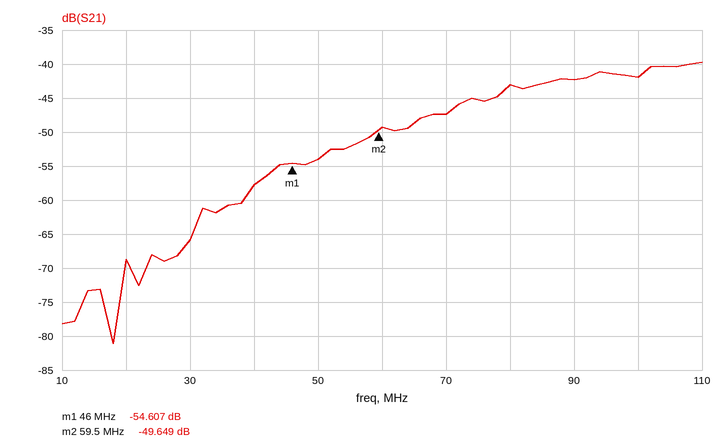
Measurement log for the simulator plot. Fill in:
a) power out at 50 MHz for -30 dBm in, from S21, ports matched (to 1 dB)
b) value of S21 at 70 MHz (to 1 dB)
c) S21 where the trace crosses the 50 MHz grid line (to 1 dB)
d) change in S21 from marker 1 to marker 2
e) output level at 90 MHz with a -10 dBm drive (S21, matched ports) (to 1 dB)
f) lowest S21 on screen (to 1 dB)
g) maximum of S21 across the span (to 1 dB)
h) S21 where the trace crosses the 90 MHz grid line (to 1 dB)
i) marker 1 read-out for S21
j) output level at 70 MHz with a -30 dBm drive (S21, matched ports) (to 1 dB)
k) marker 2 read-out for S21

-84 dBm
-47 dB
-54 dB
4.958 dB
-52 dBm
-81 dB
-40 dB
-42 dB
-54.607 dB
-77 dBm
-49.649 dB
